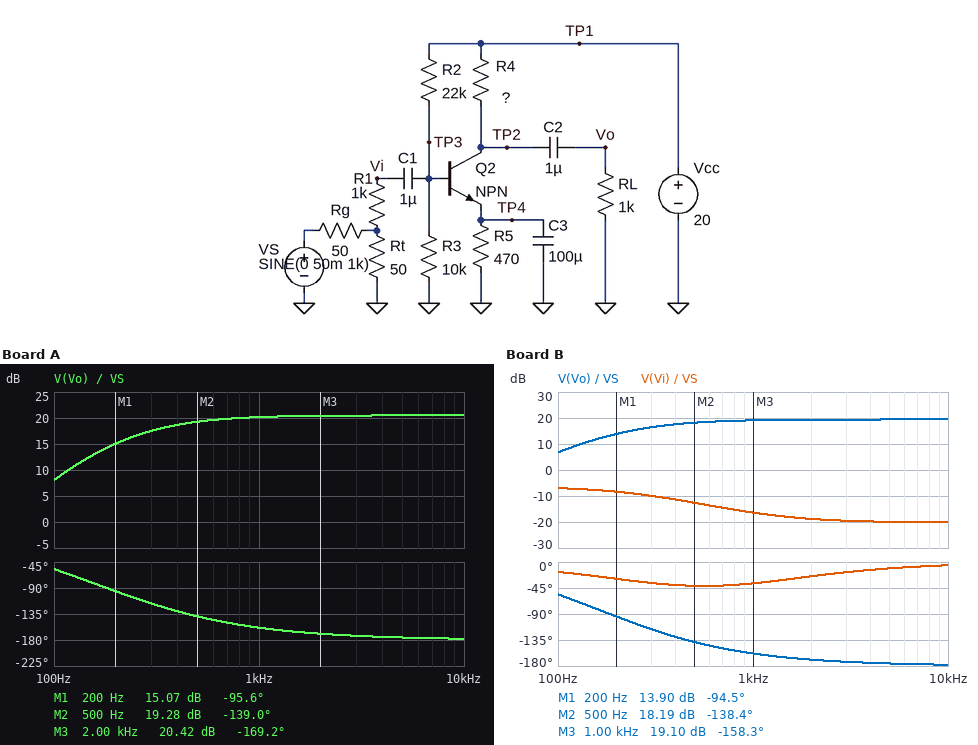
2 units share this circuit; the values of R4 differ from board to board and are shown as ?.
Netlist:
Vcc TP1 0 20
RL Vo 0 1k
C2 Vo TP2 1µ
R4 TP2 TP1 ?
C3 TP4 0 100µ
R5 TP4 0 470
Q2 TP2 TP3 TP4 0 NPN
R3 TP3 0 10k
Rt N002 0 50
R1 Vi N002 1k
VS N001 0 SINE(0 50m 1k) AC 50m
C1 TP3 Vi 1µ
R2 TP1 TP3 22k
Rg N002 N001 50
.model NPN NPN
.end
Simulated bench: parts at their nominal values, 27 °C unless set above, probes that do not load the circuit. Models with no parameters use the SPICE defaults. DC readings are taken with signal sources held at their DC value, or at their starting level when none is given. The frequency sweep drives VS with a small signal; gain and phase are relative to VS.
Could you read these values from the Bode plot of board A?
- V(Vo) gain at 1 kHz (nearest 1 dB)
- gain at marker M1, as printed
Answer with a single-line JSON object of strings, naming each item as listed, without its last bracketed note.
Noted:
{"V(Vo) gain at 1 kHz": "20 dB", "gain at marker M1, as printed": "15.07 dB"}
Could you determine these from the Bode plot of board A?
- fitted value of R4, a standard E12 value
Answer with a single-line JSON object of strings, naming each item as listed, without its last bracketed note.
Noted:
{"fitted value of R4, a standard E12 value": "390 Ω"}
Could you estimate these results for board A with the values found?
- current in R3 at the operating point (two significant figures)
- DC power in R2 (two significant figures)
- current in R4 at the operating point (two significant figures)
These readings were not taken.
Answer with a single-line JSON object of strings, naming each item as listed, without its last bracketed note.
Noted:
{"current in R3 at the operating point": "560 µA", "DC power in R2": "9.5 mW", "current in R4 at the operating point": "10 mA"}
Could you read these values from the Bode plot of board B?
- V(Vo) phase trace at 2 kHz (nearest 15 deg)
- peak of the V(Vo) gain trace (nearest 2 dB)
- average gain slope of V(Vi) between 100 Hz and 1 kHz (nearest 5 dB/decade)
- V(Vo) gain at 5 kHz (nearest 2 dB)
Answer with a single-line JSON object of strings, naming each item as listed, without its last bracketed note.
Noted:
{"V(Vo) phase trace at 2 kHz": "-165 deg", "peak of the V(Vo) gain trace": "20 dB", "average gain slope of V(Vi) between 100 Hz and 1 kHz": "-10 dB/decade", "V(Vo) gain at 5 kHz": "20 dB"}
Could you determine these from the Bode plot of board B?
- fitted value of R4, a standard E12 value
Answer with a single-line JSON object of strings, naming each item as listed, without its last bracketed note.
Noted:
{"fitted value of R4, a standard E12 value": "330 Ω"}
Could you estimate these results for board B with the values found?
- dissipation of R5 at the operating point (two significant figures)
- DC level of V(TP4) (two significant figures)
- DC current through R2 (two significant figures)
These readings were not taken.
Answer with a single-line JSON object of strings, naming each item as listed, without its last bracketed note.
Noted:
{"dissipation of R5 at the operating point": "48 mW", "DC level of V(TP4)": "4.7 V", "DC current through R2": "660 µA"}
